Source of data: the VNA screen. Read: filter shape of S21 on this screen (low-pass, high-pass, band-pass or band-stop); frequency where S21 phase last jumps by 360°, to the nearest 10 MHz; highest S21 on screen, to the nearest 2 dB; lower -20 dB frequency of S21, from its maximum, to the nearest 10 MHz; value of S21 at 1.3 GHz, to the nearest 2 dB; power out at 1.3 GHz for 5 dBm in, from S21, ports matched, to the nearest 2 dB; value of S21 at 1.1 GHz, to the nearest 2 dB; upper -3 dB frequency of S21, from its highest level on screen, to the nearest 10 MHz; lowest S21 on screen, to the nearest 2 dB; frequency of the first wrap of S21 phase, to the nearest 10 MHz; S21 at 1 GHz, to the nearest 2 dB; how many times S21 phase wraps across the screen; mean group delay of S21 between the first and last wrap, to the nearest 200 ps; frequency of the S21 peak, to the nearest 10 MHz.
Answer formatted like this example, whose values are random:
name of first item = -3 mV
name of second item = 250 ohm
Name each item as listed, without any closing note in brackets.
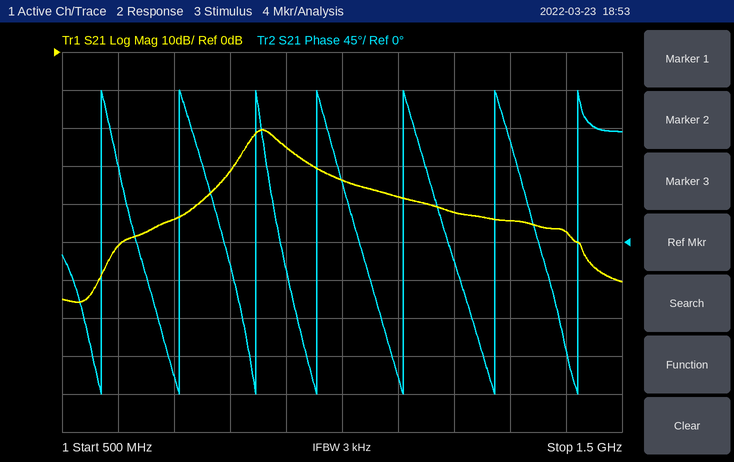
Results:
filter shape of S21 on this screen = band-pass
frequency where S21 phase last jumps by 360°, to the nearest 10 MHz = 1.42 GHz
highest S21 on screen, to the nearest 2 dB = -20 dB
lower -20 dB frequency of S21, from its maximum, to the nearest 10 MHz = 740 MHz
value of S21 at 1.3 GHz, to the nearest 2 dB = -44 dB
power out at 1.3 GHz for 5 dBm in, from S21, ports matched, to the nearest 2 dB = -40 dBm
value of S21 at 1.1 GHz, to the nearest 2 dB = -38 dB
upper -3 dB frequency of S21, from its highest level on screen, to the nearest 10 MHz = 890 MHz
lowest S21 on screen, to the nearest 2 dB = -66 dB
frequency of the first wrap of S21 phase, to the nearest 10 MHz = 570 MHz
S21 at 1 GHz, to the nearest 2 dB = -34 dB
how many times S21 phase wraps across the screen = 7
mean group delay of S21 between the first and last wrap, to the nearest 200 ps = 7.0 ns
frequency of the S21 peak, to the nearest 10 MHz = 860 MHz
